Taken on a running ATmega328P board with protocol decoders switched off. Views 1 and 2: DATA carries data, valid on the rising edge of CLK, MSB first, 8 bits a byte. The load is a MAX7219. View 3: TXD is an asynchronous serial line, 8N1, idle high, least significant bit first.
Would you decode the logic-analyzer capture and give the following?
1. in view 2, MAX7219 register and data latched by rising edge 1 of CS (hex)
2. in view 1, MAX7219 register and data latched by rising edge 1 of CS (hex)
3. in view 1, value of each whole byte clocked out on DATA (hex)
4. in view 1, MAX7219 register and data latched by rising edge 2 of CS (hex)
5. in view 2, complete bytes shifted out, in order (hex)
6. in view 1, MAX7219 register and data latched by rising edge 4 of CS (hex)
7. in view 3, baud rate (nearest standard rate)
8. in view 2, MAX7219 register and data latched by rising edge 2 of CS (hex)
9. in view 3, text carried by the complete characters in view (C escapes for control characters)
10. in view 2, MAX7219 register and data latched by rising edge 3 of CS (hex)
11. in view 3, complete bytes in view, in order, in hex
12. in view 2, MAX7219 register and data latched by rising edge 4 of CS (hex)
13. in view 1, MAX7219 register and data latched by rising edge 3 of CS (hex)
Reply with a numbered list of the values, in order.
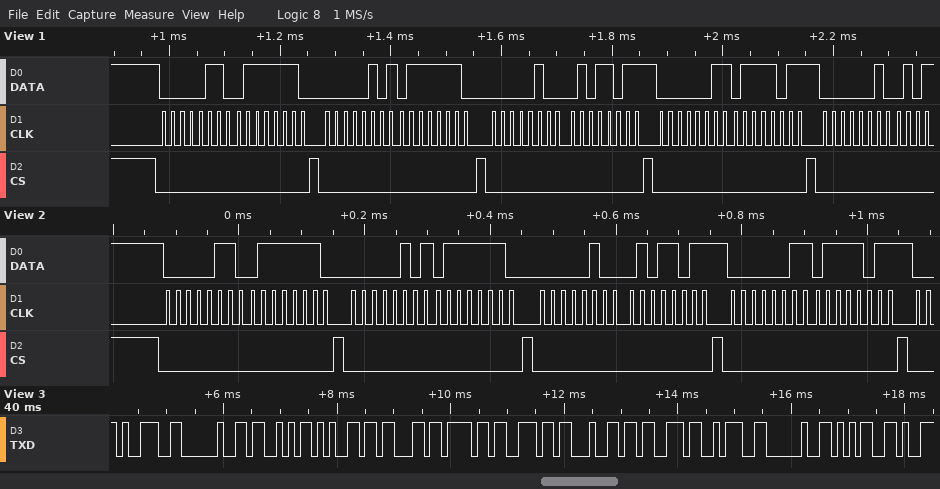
1. register 0x6, data 0x7E
2. register 0x6, data 0x7E
3. 06 7E 05 7E 04 5B 03 7B 02
4. register 0x5, data 0x7E
5. 0x06 0x7E 0x05 0x7E 0x04 0x5B 0x03 0x7B
6. register 0x3, data 0x7B
7. 9600 baud
8. register 0x5, data 0x7E
9. "9 Seconds: 5"
10. register 0x4, data 0x5B
11. 39 20 53 65 63 6F 6E 64 73 3A 20 35
12. register 0x3, data 0x7B
13. register 0x4, data 0x5B
